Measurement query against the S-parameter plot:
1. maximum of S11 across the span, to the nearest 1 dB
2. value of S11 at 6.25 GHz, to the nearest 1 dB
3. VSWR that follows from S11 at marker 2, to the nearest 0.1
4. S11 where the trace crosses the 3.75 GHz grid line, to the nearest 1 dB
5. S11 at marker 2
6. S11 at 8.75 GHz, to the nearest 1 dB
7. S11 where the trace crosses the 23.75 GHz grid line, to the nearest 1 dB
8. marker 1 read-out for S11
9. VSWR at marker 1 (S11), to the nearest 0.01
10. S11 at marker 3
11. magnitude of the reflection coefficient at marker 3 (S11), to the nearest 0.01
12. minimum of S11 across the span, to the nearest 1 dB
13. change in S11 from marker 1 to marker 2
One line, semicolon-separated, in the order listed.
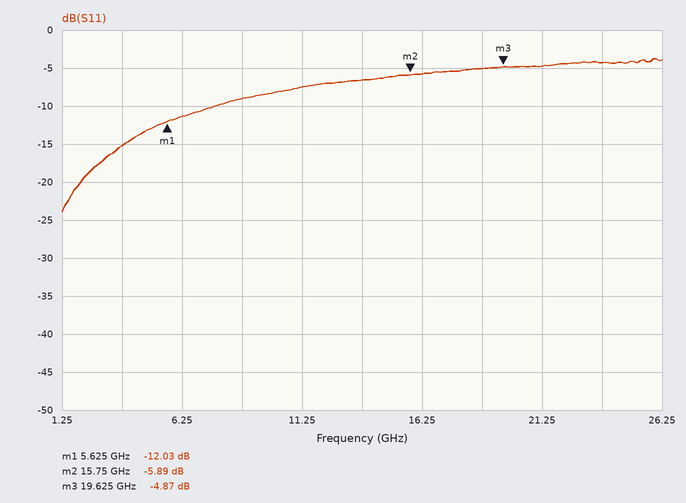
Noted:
-4 dB; -11 dB; 3.1; -15 dB; -5.89 dB; -9 dB; -4 dB; -12.03 dB; 1.67; -4.87 dB; 0.57; -24 dB; 6.14 dB
